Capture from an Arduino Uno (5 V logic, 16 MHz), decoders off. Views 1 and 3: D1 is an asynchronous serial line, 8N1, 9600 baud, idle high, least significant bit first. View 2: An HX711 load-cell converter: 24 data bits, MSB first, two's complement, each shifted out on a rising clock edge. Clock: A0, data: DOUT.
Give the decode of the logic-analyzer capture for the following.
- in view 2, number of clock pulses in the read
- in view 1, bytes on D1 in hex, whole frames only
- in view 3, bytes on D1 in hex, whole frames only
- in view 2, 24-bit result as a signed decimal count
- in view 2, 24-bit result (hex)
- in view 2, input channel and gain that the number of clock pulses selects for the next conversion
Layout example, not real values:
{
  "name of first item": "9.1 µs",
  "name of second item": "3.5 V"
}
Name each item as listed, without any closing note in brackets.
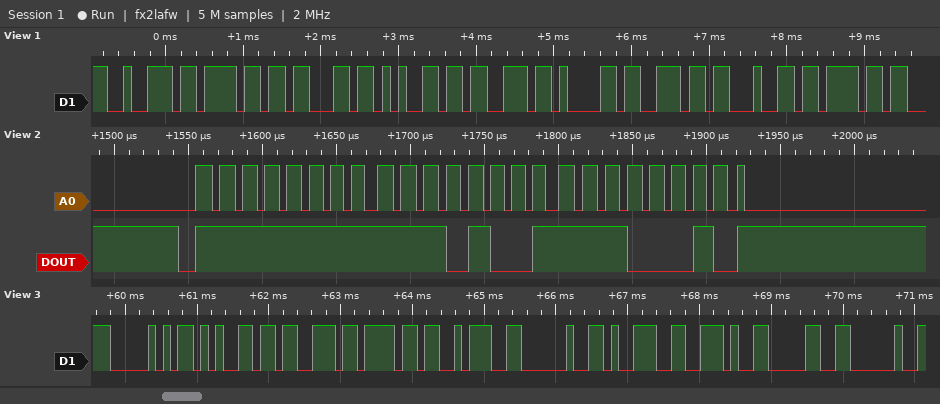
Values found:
{
  "in view 2, number of clock pulses in the read": "25",
  "in view 1, bytes on D1 in hex, whole frames only": "72 6F 63 65 73 61 6E 64 6F",
  "in view 3, bytes on D1 in hex, whole frames only": "50 65 73 6F 3A 20 39 2E 30 20",
  "in view 2, 24-bit result as a signed decimal count": "-5662",
  "in view 2, 24-bit result": "0xFFE9E2",
  "in view 2, input channel and gain that the number of clock pulses selects for the next conversion": "channel A, gain 128"
}
